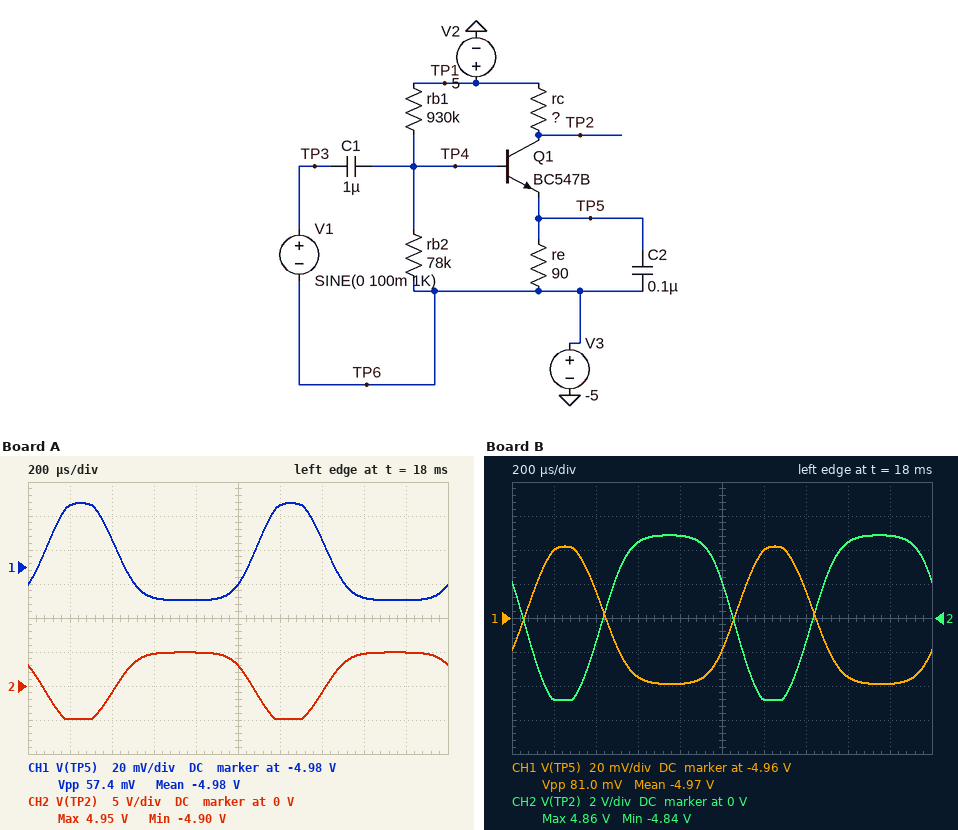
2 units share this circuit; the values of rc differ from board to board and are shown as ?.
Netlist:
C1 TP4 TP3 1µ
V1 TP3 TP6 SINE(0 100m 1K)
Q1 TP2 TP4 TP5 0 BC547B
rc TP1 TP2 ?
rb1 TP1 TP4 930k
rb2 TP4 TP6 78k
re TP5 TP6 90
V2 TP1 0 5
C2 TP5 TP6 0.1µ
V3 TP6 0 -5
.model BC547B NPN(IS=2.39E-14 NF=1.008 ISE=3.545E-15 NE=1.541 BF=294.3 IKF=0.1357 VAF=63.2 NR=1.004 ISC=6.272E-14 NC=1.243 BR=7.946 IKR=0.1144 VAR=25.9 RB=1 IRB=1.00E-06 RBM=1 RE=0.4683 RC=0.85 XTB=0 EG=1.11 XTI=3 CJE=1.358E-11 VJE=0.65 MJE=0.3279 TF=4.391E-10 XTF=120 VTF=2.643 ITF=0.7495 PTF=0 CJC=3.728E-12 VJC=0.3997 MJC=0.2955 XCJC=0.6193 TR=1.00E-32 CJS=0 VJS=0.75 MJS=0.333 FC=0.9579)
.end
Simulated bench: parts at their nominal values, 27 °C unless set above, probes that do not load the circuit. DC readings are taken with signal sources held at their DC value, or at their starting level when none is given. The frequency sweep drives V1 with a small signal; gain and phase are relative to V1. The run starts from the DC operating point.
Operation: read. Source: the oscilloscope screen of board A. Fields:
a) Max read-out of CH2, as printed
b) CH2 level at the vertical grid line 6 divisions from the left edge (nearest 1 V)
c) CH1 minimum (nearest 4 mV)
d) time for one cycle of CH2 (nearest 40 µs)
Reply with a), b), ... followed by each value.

a) 4.95 V
b) -5 V
c) -5.000 V
d) 1.00 ms
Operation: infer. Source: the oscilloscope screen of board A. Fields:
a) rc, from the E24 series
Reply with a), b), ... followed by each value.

a) 16 kΩ
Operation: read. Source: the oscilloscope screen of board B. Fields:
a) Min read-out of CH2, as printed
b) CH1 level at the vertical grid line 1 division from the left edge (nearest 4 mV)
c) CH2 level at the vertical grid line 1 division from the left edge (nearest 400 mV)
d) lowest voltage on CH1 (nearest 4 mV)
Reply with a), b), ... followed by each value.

a) -4.84 V
b) -4.920 V
c) -4.8 V
d) -5.000 V
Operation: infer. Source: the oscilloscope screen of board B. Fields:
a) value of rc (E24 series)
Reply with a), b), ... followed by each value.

a) 11 kΩ
